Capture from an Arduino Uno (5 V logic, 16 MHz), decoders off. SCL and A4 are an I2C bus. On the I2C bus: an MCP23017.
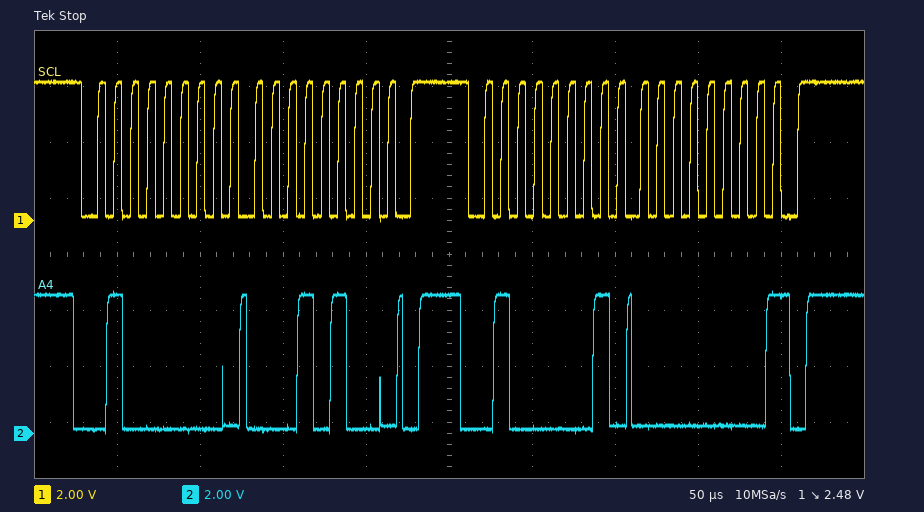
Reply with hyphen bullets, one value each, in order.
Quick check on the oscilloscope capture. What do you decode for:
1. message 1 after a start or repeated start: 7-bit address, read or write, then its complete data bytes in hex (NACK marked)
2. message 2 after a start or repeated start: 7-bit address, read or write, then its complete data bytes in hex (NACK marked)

- 0x20 write: 14
- 0x20 read: 00 NACK
